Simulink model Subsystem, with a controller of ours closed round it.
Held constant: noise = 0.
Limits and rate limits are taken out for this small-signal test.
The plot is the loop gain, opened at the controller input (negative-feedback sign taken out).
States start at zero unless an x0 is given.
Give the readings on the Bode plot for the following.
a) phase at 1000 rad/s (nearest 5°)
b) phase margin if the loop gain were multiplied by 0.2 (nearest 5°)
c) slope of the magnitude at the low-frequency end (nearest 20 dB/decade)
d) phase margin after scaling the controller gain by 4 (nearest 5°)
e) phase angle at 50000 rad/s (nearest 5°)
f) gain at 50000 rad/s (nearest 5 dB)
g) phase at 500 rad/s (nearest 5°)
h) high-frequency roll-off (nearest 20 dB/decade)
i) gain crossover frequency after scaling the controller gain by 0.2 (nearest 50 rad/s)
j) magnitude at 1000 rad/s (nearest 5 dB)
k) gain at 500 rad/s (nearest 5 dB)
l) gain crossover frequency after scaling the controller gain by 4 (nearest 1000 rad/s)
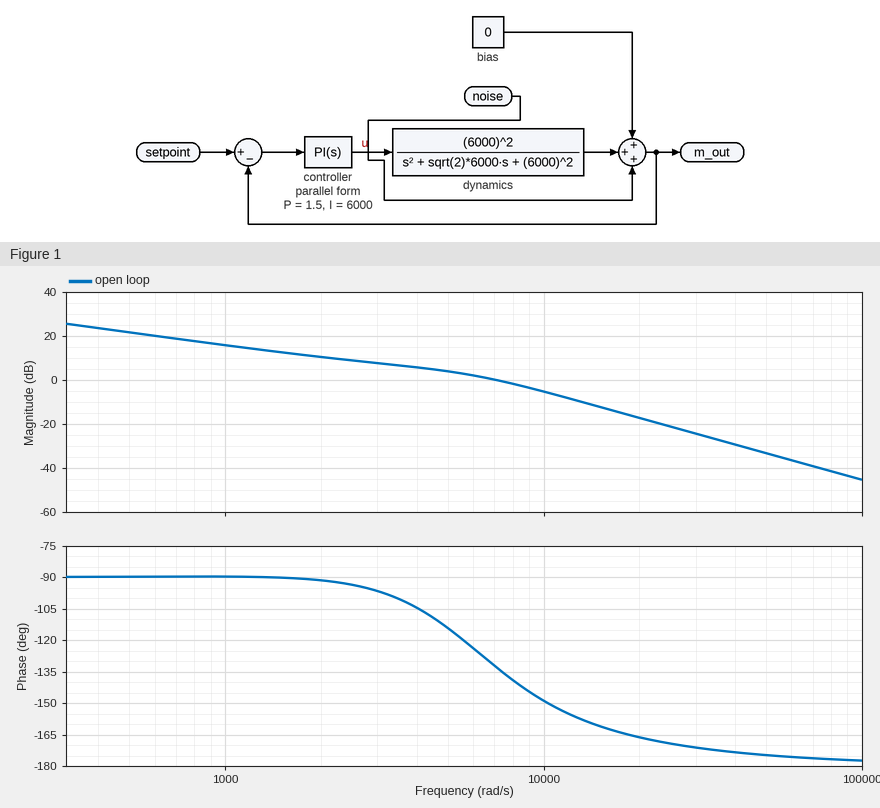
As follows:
-90°
90°
-20 dB/decade
20°
-175°
-35 dB
-90°
-40 dB/decade
1250 rad/s
15 dB
20 dB
15000 rad/s
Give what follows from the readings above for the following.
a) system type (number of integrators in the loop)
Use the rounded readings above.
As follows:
1
